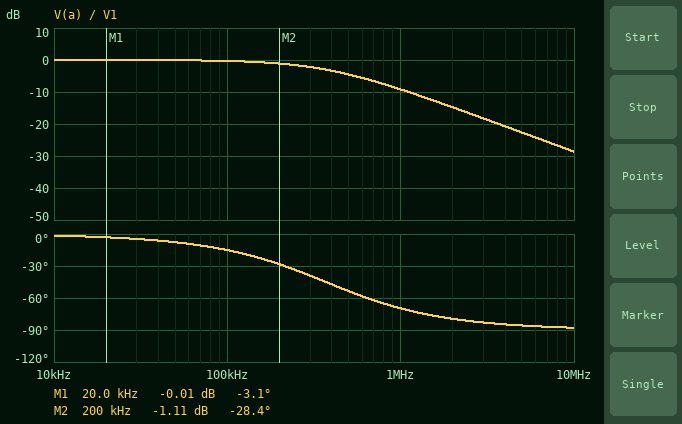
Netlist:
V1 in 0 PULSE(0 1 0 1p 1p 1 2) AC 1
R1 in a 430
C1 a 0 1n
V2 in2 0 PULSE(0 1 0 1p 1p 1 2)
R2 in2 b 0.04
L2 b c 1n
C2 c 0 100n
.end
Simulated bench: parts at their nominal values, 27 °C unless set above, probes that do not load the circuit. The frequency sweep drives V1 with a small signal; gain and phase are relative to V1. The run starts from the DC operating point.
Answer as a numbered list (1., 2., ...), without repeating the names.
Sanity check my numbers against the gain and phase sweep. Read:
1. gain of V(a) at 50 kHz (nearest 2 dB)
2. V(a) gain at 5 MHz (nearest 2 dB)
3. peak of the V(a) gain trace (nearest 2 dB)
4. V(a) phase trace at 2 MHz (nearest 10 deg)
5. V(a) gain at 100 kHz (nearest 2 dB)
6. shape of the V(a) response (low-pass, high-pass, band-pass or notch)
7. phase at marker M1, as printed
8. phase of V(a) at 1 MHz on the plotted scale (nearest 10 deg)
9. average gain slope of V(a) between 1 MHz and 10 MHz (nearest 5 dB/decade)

1. 0 dB
2. -22 dB
3. 0 dB
4. -80 deg
5. 0 dB
6. low-pass
7. -3.1 deg
8. -70 deg
9. -20 dB/decade
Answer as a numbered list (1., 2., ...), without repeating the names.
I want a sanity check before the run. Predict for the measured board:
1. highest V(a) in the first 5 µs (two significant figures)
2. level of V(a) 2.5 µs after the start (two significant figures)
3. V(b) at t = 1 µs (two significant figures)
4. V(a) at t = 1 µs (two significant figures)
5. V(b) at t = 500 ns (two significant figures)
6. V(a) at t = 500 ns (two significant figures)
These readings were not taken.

1. 1.0 V
2. 1.0 V
3. 1.0 V
4. 900 mV
5. 1.0 V
6. 690 mV
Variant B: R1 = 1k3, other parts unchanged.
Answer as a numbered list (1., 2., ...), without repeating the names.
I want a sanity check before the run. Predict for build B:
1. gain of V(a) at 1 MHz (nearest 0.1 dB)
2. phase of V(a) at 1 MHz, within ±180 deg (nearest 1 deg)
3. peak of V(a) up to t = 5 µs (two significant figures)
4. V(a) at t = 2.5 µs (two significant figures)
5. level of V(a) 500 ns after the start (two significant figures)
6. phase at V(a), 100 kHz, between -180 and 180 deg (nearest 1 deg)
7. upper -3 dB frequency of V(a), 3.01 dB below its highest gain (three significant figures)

1. -18.3 dB
2. -83 deg
3. 980 mV
4. 850 mV
5. 320 mV
6. -39 deg
7. 122 kHz
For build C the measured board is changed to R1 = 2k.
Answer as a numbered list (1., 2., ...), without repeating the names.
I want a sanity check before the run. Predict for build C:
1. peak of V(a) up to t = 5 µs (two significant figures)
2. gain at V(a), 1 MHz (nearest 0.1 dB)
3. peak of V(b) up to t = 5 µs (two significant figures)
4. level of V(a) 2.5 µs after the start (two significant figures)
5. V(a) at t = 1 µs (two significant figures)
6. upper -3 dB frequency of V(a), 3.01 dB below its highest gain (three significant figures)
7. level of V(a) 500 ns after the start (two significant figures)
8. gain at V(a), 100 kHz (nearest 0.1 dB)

1. 920 mV
2. -22.0 dB
3. 1.2 V
4. 710 mV
5. 390 mV
6. 79.6 kHz
7. 220 mV
8. -4.1 dB
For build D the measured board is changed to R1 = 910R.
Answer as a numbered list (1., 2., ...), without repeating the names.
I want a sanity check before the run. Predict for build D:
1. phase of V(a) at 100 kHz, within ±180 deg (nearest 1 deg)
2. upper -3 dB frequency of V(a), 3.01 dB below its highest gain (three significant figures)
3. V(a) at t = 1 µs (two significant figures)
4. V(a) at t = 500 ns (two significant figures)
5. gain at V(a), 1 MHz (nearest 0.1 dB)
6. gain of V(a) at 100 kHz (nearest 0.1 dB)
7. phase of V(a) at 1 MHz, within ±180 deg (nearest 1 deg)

1. -30 deg
2. 175 kHz
3. 670 mV
4. 420 mV
5. -15.3 dB
6. -1.2 dB
7. -80 deg
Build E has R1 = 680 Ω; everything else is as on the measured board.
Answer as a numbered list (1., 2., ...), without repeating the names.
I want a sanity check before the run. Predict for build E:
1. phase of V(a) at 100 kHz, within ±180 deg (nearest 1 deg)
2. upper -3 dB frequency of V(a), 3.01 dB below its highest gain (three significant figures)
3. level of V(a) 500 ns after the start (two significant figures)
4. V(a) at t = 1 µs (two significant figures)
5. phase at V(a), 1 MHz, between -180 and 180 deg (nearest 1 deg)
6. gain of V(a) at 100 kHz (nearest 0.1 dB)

1. -23 deg
2. 234 kHz
3. 520 mV
4. 770 mV
5. -77 deg
6. -0.7 dB
